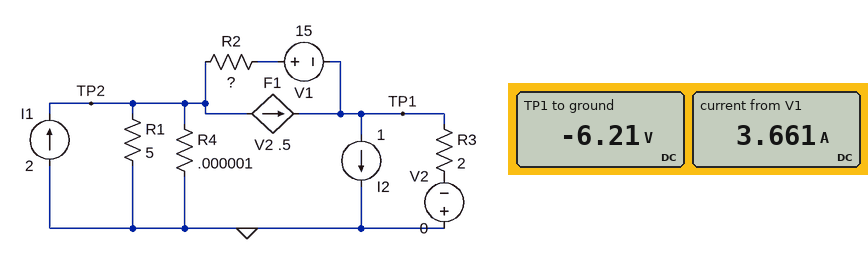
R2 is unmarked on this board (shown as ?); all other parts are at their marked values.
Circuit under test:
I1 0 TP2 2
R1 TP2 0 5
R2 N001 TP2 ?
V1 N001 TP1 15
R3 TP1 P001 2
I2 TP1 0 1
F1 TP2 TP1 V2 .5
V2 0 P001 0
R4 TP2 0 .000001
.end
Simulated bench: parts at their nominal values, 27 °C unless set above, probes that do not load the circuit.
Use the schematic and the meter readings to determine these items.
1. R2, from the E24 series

2.4 Ω
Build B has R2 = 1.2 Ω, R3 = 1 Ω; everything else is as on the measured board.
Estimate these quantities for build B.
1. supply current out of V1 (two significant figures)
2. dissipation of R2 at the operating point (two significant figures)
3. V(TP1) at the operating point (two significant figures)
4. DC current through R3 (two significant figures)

7.7 A
71 W
-5.8 V
5.8 A
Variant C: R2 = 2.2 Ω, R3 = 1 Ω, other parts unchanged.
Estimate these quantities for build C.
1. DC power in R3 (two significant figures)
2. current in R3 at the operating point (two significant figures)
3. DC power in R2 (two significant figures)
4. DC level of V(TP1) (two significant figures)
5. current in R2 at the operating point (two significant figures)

16 W
4.0 A
55 W
-4.0 V
5.0 A
